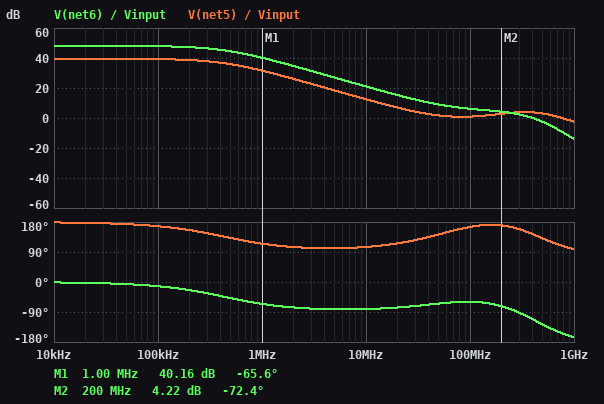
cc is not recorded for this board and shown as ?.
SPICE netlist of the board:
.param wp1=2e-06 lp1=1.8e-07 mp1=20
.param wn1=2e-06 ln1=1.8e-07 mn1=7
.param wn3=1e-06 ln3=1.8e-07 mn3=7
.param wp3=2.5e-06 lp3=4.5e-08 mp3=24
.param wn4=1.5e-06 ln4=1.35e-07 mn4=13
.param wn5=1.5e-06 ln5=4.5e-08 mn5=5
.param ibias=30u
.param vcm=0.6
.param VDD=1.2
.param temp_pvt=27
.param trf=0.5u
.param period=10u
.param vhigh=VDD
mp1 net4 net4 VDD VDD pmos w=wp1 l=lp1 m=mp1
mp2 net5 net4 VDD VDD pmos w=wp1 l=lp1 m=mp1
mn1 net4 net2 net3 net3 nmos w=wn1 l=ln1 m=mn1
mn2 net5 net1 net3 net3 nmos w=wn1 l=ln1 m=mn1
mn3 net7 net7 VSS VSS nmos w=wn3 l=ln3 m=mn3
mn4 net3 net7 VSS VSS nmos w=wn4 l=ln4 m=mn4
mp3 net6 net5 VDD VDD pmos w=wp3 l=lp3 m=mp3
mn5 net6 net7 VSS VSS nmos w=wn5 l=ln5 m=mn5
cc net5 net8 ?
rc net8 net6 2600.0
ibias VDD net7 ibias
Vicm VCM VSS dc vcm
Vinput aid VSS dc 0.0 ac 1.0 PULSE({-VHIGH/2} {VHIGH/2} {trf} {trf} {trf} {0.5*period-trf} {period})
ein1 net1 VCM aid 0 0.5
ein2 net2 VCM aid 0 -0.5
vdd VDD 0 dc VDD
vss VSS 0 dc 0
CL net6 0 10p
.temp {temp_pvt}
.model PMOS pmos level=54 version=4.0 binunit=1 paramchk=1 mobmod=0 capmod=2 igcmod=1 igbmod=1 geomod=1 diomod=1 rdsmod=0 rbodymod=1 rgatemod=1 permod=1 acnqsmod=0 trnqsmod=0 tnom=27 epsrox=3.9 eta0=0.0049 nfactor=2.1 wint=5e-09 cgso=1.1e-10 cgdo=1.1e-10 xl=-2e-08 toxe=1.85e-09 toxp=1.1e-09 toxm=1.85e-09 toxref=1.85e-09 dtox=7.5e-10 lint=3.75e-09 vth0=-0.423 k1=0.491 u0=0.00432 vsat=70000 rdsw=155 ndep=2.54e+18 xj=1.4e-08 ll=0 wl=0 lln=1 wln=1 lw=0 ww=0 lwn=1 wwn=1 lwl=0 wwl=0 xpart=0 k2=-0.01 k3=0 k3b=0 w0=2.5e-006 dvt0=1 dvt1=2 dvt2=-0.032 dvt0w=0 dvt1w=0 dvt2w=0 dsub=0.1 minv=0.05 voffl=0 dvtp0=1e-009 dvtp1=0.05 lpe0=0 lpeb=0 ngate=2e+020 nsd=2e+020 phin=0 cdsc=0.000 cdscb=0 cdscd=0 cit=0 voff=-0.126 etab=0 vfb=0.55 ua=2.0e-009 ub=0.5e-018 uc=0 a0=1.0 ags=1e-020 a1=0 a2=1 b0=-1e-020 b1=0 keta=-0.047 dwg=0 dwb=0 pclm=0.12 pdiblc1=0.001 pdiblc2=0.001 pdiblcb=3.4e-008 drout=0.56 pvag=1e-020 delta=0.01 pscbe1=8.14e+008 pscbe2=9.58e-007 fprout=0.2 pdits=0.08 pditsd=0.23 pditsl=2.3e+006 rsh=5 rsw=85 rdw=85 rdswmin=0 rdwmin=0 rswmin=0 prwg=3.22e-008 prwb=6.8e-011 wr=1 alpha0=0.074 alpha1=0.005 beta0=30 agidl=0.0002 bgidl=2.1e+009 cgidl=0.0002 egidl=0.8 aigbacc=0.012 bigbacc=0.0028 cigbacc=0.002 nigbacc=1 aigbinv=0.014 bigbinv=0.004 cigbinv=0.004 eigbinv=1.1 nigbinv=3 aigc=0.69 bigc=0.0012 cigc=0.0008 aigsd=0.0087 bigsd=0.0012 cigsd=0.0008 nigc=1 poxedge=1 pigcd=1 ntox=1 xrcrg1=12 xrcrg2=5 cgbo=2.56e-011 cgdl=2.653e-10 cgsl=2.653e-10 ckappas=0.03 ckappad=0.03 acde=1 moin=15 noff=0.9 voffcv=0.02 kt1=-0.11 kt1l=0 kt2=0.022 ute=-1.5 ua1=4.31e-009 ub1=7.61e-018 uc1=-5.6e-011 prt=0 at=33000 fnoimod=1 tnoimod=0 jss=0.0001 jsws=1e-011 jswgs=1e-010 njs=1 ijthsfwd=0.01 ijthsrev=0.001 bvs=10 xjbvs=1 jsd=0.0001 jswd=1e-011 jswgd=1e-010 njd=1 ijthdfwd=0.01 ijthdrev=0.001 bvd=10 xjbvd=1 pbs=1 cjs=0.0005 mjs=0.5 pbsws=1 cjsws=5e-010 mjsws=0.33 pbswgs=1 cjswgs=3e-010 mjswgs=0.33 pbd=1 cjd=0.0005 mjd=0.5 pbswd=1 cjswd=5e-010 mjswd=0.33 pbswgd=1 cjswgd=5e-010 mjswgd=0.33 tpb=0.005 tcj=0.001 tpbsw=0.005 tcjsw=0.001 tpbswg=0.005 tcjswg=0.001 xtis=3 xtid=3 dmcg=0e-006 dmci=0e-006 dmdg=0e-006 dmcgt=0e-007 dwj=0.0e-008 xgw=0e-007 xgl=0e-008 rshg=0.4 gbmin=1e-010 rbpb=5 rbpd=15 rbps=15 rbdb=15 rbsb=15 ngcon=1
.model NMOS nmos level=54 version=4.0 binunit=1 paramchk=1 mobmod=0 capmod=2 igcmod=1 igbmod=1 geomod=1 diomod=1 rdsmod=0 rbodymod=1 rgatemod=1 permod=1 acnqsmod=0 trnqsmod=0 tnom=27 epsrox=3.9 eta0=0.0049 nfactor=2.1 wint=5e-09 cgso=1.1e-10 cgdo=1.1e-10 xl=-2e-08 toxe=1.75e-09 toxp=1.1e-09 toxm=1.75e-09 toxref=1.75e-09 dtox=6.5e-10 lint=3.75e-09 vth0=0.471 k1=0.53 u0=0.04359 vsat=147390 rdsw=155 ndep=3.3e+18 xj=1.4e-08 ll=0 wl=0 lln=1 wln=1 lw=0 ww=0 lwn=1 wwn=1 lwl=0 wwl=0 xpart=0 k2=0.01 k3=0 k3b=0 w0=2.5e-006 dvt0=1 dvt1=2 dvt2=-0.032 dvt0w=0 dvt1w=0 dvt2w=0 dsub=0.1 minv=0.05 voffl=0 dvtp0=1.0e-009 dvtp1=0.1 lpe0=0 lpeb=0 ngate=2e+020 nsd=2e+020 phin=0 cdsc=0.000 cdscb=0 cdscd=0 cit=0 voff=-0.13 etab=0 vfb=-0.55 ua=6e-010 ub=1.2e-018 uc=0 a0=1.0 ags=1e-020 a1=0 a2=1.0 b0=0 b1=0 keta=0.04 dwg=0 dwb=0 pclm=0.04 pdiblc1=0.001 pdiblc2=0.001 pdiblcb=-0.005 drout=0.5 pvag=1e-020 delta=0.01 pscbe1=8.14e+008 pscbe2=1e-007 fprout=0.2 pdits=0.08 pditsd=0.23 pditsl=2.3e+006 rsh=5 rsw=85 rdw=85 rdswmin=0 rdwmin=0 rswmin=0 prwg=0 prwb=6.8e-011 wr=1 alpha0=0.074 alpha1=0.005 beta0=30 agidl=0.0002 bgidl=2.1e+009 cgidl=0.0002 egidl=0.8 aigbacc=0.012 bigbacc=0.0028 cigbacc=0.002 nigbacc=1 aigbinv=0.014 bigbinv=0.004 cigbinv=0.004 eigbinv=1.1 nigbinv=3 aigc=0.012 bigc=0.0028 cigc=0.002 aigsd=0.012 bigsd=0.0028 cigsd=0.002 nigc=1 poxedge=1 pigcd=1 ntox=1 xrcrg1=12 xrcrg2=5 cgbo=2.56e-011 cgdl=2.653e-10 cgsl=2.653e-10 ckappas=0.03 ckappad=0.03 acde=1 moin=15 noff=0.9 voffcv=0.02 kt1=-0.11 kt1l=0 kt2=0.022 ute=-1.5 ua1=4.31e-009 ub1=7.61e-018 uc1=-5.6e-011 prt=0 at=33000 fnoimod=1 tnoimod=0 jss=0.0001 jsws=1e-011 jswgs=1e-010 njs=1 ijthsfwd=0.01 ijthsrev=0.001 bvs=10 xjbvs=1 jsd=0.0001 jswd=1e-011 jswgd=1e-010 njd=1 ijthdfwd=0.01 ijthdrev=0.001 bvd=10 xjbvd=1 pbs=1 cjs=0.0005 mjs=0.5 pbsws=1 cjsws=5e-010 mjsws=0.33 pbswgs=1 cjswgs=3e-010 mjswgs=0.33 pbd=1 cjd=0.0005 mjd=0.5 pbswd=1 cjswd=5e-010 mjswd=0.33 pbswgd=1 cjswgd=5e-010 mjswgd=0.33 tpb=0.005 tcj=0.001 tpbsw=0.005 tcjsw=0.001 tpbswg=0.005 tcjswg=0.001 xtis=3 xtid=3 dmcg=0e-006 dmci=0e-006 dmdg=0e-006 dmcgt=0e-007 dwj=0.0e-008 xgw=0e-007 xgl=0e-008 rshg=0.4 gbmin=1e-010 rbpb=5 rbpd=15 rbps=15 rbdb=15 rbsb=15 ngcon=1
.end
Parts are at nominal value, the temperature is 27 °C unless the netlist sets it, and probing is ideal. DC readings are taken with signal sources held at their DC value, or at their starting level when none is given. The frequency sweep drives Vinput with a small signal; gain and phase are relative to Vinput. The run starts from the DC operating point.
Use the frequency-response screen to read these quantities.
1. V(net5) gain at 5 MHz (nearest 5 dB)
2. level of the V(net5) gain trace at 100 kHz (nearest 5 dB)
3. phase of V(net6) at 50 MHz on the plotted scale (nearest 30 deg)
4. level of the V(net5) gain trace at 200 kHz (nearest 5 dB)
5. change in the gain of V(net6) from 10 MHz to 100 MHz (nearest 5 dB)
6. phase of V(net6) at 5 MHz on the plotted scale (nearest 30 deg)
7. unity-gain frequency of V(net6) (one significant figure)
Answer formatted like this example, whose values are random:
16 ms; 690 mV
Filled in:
20 dB; 40 dB; -60 deg; 40 dB; -15 dB; -90 deg; 400 MHz
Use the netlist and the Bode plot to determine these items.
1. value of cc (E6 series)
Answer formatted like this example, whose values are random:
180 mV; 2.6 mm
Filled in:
1 pF
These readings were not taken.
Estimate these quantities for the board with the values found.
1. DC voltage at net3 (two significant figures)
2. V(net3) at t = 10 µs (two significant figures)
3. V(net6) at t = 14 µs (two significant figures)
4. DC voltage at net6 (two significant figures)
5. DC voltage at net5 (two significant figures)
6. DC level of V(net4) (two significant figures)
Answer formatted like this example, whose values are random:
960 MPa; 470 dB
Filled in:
150 mV; 400 mV; 1.2 V; 940 mV; 700 mV; 700 mV
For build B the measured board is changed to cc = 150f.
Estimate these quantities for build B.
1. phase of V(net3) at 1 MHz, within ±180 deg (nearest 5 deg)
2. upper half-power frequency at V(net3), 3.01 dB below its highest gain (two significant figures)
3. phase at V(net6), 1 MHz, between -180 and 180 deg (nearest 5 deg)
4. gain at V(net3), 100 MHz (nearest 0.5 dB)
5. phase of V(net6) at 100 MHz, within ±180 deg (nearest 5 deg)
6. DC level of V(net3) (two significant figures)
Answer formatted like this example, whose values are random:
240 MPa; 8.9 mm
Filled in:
160 deg; 2.3 MHz; -25 deg; -34.5 dB; -105 deg; 150 mV
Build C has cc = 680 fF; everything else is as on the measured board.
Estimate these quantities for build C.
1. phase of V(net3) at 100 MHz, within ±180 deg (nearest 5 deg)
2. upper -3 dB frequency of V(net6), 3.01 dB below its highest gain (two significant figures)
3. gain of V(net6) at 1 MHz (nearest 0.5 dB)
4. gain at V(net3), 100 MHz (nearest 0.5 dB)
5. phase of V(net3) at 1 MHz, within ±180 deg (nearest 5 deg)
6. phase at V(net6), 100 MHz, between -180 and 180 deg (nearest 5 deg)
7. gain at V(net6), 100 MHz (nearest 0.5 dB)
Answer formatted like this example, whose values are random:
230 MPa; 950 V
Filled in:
-170 deg; 630 kHz; 42.5 dB; -43.5 dB; 125 deg; -70 deg; 7.0 dB
